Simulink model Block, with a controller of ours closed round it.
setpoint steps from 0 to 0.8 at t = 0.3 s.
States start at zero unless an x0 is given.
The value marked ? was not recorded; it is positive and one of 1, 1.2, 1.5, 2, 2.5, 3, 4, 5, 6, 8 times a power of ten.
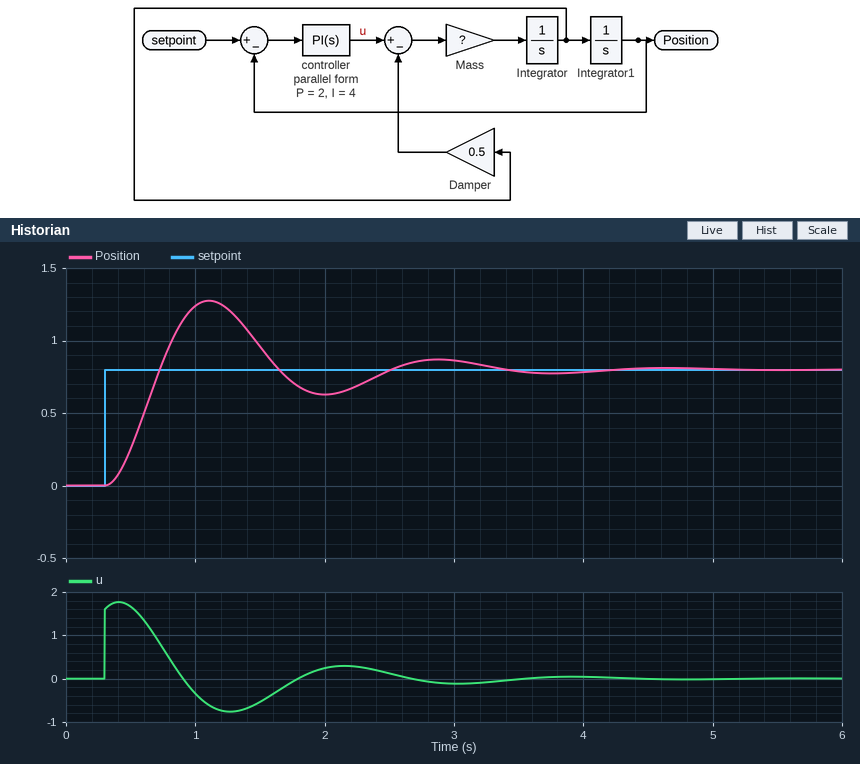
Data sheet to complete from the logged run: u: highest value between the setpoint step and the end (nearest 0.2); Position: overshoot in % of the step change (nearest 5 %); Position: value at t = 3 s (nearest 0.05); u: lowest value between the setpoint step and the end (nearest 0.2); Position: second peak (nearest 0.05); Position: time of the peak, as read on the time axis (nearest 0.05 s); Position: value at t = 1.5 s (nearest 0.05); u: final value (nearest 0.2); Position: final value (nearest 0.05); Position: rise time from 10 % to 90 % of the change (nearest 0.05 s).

1.8
60 %
0.85
-0.8
0.85
1.10 s
0.95
0.0
0.80
0.30 s
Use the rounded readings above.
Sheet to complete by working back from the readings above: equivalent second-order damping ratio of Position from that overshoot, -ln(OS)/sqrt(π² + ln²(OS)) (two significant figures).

0.16
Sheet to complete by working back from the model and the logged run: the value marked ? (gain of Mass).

10
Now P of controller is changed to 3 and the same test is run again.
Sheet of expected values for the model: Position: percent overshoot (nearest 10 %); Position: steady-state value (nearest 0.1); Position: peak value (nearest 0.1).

50 %
0.8
1.2
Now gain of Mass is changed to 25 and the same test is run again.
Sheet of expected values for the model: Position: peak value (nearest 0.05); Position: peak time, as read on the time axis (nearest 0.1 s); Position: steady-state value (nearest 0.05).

1.05
1.0 s
0.80
